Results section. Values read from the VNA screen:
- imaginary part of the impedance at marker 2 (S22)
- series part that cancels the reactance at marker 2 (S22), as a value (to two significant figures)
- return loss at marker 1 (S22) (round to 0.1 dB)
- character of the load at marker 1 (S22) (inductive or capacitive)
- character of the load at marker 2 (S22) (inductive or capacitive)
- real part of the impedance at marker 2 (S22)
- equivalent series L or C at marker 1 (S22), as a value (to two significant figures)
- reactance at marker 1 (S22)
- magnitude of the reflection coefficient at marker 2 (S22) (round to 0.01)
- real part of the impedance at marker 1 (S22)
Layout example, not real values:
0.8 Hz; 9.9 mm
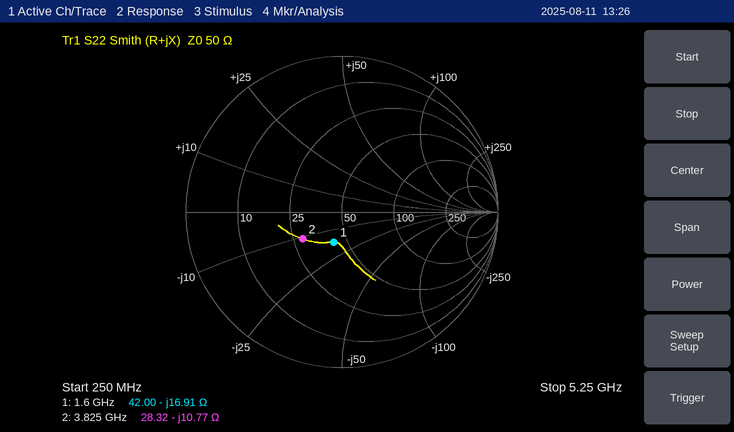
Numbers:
-10.77 Ω; 450 pH; 14.0 dB; capacitive; capacitive; 28.32 Ω; 5.9 pF; -16.91 Ω; 0.31; 42.00 Ω
